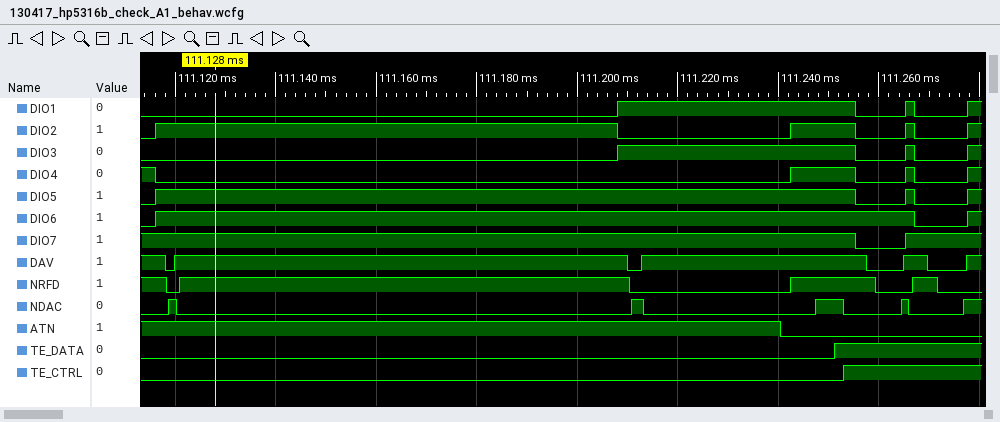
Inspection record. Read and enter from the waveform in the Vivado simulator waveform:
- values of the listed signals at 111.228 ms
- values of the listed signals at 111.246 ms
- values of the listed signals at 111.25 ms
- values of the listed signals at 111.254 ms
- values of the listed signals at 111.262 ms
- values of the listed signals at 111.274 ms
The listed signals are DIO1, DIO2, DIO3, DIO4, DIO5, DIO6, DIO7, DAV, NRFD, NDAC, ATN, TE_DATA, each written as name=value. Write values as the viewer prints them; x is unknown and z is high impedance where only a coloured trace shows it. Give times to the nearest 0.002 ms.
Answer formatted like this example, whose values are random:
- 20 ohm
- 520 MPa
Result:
- DIO1=1, DIO2=0, DIO3=1, DIO4=0, DIO5=1, DIO6=1, DIO7=1, DAV=1, NRFD=0, NDAC=0, ATN=1, TE_DATA=0
- DIO1=1, DIO2=1, DIO3=1, DIO4=1, DIO5=1, DIO6=1, DIO7=1, DAV=1, NRFD=1, NDAC=0, ATN=0, TE_DATA=0
- DIO1=1, DIO2=1, DIO3=1, DIO4=1, DIO5=1, DIO6=1, DIO7=1, DAV=1, NRFD=1, NDAC=1, ATN=0, TE_DATA=0
- DIO1=1, DIO2=1, DIO3=1, DIO4=1, DIO5=1, DIO6=1, DIO7=1, DAV=1, NRFD=1, NDAC=0, ATN=0, TE_DATA=1
- DIO1=0, DIO2=0, DIO3=0, DIO4=0, DIO5=0, DIO6=1, DIO7=0, DAV=0, NRFD=0, NDAC=0, ATN=0, TE_DATA=1
- DIO1=0, DIO2=0, DIO3=0, DIO4=0, DIO5=0, DIO6=0, DIO7=1, DAV=0, NRFD=0, NDAC=0, ATN=0, TE_DATA=1
